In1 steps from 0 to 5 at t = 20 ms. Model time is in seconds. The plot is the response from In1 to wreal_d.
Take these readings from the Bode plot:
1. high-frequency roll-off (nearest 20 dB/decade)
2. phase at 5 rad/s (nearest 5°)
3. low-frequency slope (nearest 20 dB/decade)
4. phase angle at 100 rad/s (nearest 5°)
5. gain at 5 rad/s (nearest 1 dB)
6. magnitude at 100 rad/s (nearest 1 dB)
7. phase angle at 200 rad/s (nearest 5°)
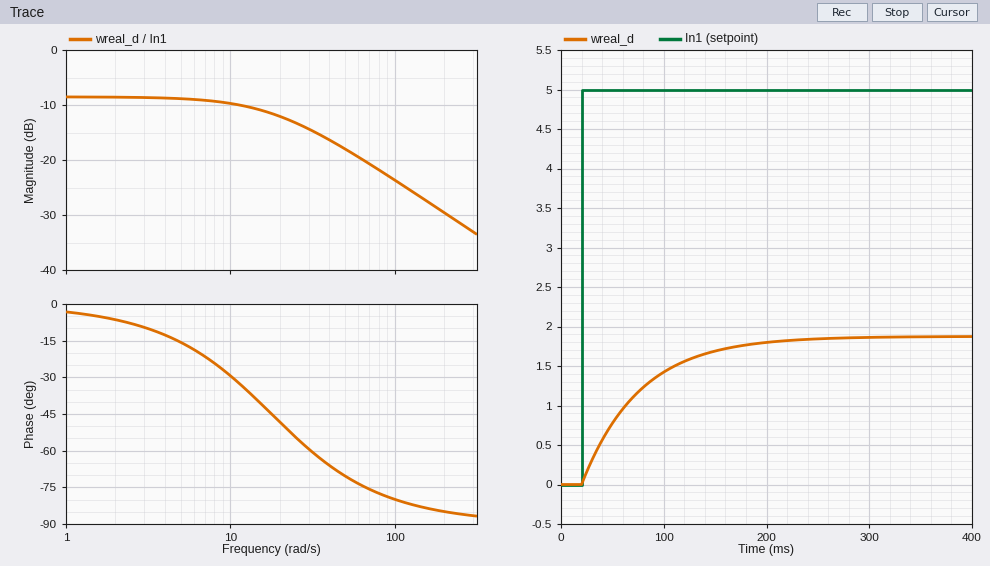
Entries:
-20 dB/decade
-15°
0 dB/decade
-80°
-9 dB
-24 dB
-85°
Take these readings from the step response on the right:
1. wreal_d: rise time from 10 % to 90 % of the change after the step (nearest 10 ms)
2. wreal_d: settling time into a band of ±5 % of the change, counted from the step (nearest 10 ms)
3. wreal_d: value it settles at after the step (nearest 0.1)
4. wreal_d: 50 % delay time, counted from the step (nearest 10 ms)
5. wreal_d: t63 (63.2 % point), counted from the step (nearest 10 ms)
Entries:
120 ms
170 ms
1.9
40 ms
60 ms
